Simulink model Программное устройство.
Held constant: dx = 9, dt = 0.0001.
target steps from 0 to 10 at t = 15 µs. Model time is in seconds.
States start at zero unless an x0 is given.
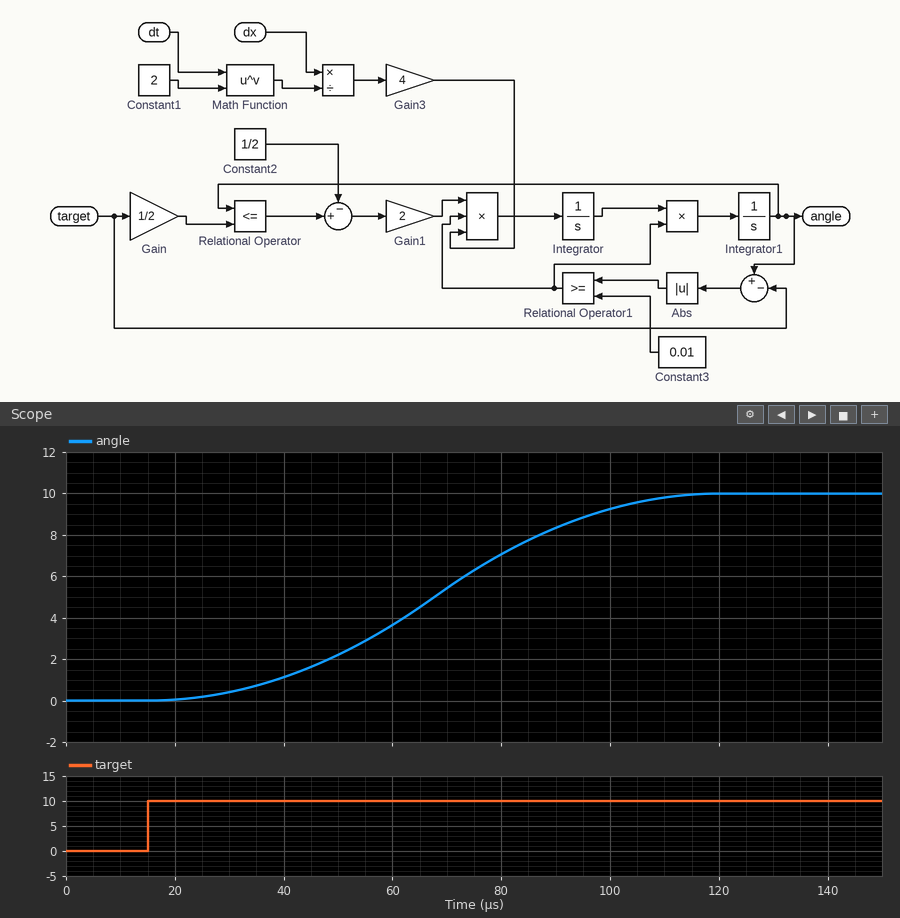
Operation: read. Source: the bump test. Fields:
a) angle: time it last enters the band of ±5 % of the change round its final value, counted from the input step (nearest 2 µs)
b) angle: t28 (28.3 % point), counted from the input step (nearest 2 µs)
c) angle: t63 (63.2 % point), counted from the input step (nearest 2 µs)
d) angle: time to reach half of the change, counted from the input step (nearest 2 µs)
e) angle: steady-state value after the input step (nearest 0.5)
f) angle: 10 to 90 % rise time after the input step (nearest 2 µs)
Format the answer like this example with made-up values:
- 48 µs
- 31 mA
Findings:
- 88 µs
- 40 µs
- 60 µs
- 52 µs
- 10.0
- 58 µs
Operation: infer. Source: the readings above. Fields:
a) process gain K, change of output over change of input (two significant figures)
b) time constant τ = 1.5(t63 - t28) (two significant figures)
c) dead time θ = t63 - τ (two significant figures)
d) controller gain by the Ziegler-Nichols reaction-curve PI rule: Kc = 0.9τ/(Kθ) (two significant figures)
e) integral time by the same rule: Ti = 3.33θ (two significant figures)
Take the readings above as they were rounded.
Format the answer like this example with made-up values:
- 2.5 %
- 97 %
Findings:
- 1.0
- 30 µs
- 30 µs
- 0.90
- 100 µs
